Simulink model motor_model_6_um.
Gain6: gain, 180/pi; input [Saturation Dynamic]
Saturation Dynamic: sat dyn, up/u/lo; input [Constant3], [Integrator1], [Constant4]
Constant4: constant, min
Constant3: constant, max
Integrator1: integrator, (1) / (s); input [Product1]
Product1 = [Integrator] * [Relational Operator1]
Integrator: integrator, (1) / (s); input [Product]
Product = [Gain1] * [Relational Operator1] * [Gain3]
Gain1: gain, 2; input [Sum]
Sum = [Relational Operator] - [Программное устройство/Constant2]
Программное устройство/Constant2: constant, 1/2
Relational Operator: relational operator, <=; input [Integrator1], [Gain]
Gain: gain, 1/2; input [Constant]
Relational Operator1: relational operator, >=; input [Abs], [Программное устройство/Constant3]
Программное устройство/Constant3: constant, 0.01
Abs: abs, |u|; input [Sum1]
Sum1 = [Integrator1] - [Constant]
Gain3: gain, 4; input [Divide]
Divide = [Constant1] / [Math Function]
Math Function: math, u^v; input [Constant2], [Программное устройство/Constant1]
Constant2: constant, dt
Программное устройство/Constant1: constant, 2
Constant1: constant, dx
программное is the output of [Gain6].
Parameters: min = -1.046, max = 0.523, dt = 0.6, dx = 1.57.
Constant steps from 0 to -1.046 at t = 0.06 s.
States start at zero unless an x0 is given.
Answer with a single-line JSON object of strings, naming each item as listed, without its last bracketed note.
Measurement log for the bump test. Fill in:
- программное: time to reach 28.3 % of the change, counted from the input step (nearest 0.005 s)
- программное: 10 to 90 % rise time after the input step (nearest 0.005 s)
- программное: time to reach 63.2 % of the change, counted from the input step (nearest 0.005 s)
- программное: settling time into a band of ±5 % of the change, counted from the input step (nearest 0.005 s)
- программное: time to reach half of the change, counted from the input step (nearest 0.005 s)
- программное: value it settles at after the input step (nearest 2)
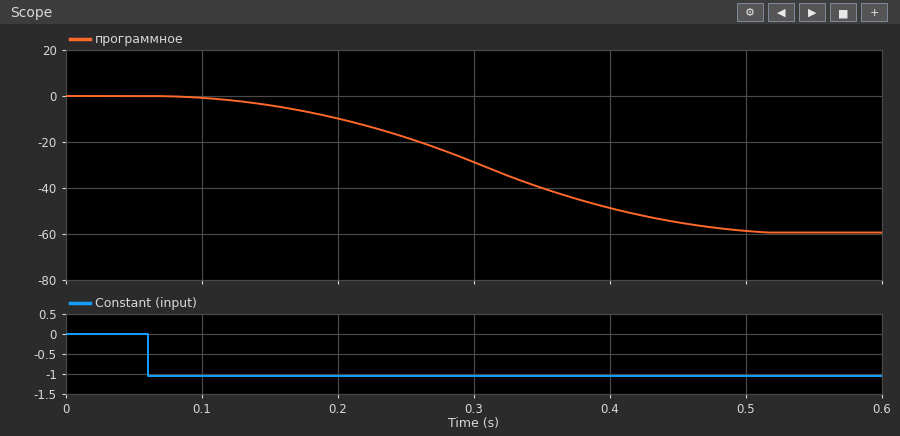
{"программное: time to reach 28.3 % of the change, counted from the input step": "0.185 s", "программное: 10 to 90 % rise time after the input step": "0.265 s", "программное: time to reach 63.2 % of the change, counted from the input step": "0.280 s", "программное: settling time into a band of ±5 % of the change, counted from the input step": "0.405 s", "программное: time to reach half of the change, counted from the input step": "0.245 s", "программное: value it settles at after the input step": "-60"}
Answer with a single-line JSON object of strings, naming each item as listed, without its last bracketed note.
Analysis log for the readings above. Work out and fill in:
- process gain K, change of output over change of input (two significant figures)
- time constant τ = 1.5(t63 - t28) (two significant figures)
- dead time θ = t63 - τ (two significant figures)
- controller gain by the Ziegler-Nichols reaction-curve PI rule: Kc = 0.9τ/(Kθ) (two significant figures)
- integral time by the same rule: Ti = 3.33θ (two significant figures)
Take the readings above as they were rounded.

{"process gain K, change of output over change of input": "57", "time constant τ = 1.5(t63 - t28)": "0.14 s", "dead time θ = t63 - τ": "0.14 s", "controller gain by the Ziegler-Nichols reaction-curve PI rule: Kc = 0.9τ/(Kθ)": "0.016", "integral time by the same rule: Ti = 3.33θ": "0.47 s"}
